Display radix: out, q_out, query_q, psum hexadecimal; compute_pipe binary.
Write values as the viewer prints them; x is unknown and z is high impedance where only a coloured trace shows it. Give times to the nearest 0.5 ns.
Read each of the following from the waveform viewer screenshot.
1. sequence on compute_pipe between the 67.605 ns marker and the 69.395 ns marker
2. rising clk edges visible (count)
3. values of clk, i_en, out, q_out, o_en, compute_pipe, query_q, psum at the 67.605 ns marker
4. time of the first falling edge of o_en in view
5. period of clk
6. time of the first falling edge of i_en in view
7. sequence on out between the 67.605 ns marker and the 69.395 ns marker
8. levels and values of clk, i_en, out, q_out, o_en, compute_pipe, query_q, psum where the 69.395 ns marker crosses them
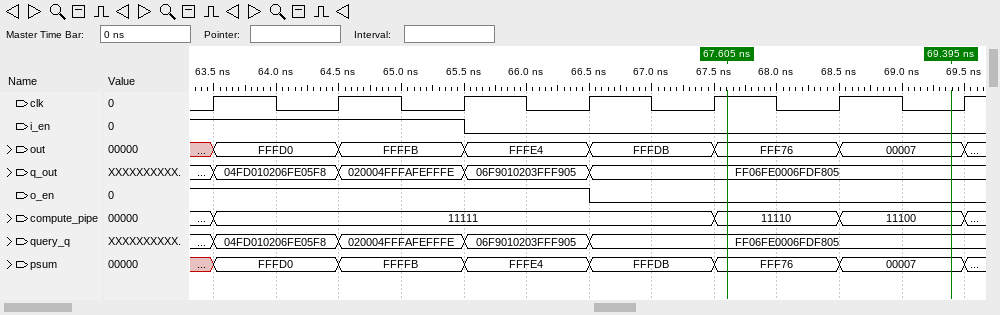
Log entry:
11110, 11100
7
clk=1, i_en=0, out=FFF76, q_out=FF06FE0006FDF805, o_en=0, compute_pipe=11110, query_q=FF06FE0006FDF805, psum=FFF76
66.5 ns
1 ns
65.5 ns
FFF76, 00007
clk=0, i_en=0, out=00007, q_out=FF06FE0006FDF805, o_en=0, compute_pipe=11100, query_q=FF06FE0006FDF805, psum=00007
